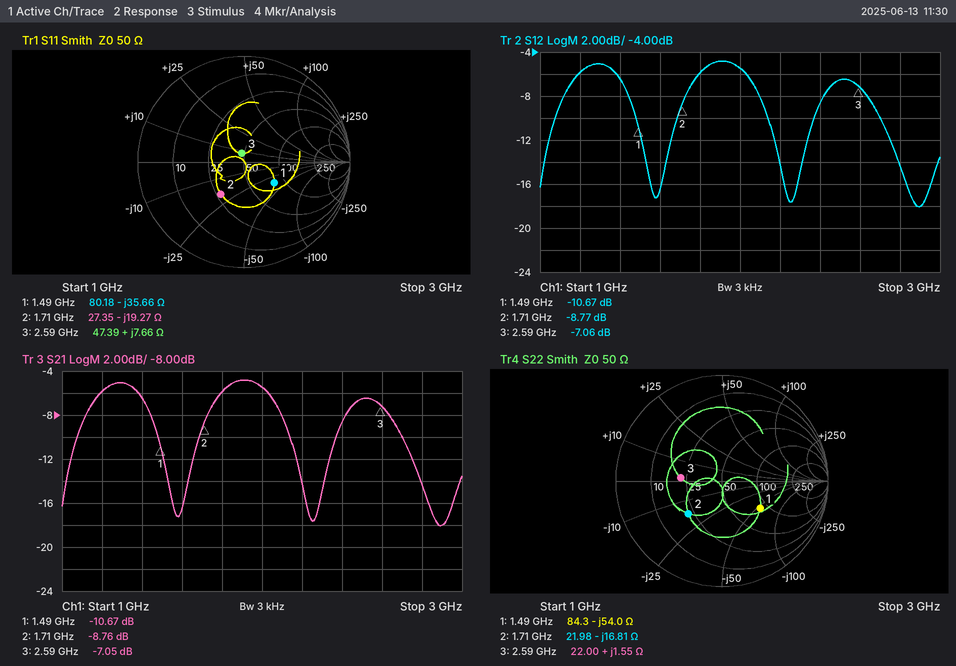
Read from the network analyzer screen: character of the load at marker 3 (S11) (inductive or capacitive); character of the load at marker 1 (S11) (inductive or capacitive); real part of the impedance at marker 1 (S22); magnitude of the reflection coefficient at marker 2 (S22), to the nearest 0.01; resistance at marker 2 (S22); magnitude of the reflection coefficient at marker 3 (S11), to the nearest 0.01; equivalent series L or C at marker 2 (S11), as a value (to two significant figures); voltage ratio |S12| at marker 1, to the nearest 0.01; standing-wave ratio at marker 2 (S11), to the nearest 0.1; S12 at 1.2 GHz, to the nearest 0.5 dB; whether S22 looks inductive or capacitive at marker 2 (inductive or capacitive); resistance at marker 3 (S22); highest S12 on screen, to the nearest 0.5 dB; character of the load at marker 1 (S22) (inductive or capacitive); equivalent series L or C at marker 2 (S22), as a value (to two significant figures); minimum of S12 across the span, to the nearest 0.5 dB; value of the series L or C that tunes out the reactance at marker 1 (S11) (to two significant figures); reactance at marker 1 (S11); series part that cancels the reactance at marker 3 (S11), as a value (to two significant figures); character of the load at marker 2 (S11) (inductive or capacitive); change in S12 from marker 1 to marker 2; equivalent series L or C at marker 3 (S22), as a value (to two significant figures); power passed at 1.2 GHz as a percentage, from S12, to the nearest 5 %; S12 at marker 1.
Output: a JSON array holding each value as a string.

["inductive", "capacitive", "84.3 Ω", "0.44", "21.98 Ω", "0.08", "4.8 pF", "0.29", "2.2", "-6.0 dB", "capacitive", "22.00 Ω", "-5.0 dB", "capacitive", "5.5 pF", "-18.0 dB", "3.8 nH", "-35.66 Ω", "8.0 pF", "capacitive", "1.90 dB", "95 pH", "25 %", "-10.67 dB"]
